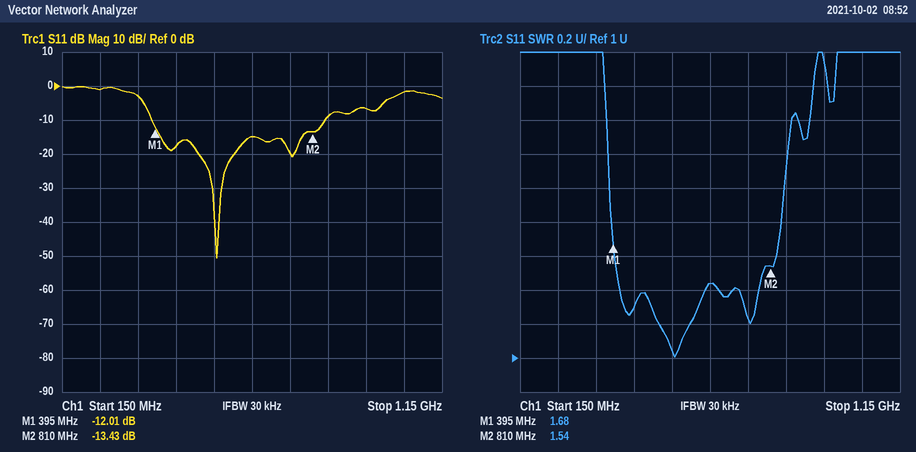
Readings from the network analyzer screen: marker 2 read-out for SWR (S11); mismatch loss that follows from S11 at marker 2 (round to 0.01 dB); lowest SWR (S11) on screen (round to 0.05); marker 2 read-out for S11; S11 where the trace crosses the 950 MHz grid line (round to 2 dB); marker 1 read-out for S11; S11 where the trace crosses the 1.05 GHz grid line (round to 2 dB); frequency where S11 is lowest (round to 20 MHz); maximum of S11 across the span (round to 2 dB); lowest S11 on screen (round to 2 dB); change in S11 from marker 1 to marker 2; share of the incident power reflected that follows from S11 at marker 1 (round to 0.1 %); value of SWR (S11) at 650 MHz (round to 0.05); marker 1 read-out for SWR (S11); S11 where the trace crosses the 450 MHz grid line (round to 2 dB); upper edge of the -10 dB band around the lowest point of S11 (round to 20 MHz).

1.54
0.20 dB
1.00
-13.43 dB
-6 dB
-12.01 dB
-2 dB
560 MHz
0 dB
-50 dB
-1.42 dB
6.3 %
1.45
1.68
-18 dB
840 MHz
